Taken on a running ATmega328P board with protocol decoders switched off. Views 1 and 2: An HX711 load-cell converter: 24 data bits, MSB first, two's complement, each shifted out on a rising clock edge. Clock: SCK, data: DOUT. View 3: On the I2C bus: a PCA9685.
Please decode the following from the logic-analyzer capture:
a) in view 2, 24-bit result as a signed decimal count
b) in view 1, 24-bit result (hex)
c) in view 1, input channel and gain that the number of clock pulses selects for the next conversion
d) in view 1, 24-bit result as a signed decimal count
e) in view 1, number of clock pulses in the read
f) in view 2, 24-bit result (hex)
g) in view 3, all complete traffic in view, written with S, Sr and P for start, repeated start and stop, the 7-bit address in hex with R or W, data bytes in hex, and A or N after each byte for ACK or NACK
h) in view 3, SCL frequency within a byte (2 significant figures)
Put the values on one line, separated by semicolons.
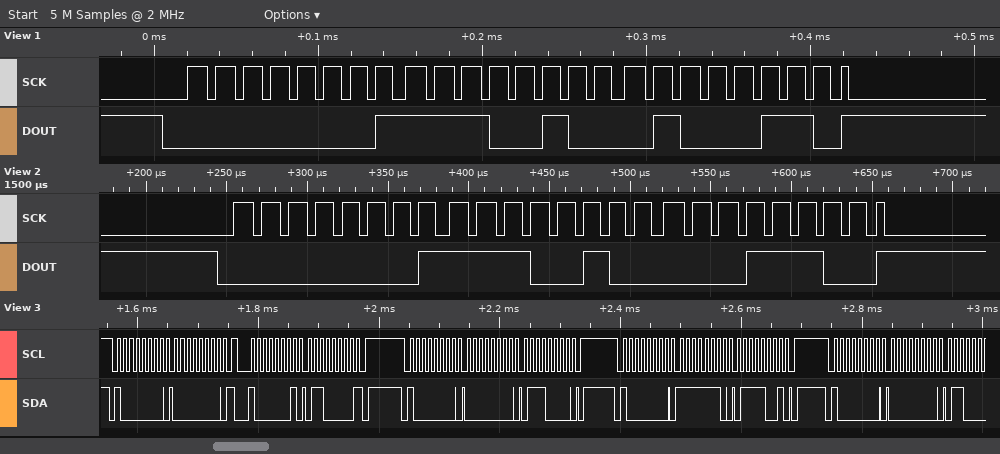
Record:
123932; 0x01E446; channel A, gain 128; 123974; 25; 0x01E41C; S 40W A 00 A Sr 40R A 60 N P S 40W A 00 A 70 A P S 40W A FE A 79 A P S 40W A 00 A; 100 kHz
